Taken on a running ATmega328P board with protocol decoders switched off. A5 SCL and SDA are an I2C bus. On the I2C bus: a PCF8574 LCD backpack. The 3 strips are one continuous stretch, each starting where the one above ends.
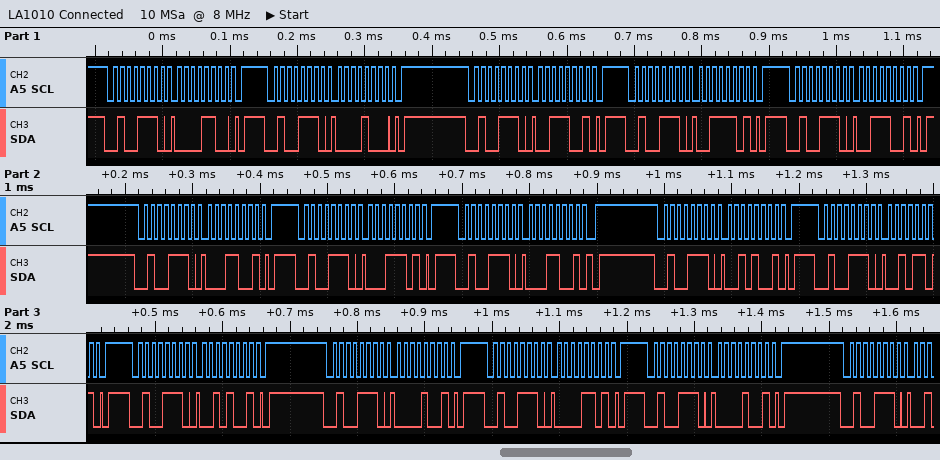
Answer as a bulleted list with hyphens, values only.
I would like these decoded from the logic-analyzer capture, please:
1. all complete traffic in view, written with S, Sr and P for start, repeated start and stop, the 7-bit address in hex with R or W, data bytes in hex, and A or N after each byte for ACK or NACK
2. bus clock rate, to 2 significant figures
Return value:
- S 27W A 0C A P S 27W A 08 A P S 27W A 39 A P S 27W A 3D A P S 27W A 39 A P S 27W A 19 A P S 27W A 1D A P S 27W A 19 A P S 27W A 29 A P S 27W A 2D A P S 27W A 29 A P S 27W A 09 A P S 27W A 0D A P S 27W A 09 A P S 27W A
- 100 kHz
